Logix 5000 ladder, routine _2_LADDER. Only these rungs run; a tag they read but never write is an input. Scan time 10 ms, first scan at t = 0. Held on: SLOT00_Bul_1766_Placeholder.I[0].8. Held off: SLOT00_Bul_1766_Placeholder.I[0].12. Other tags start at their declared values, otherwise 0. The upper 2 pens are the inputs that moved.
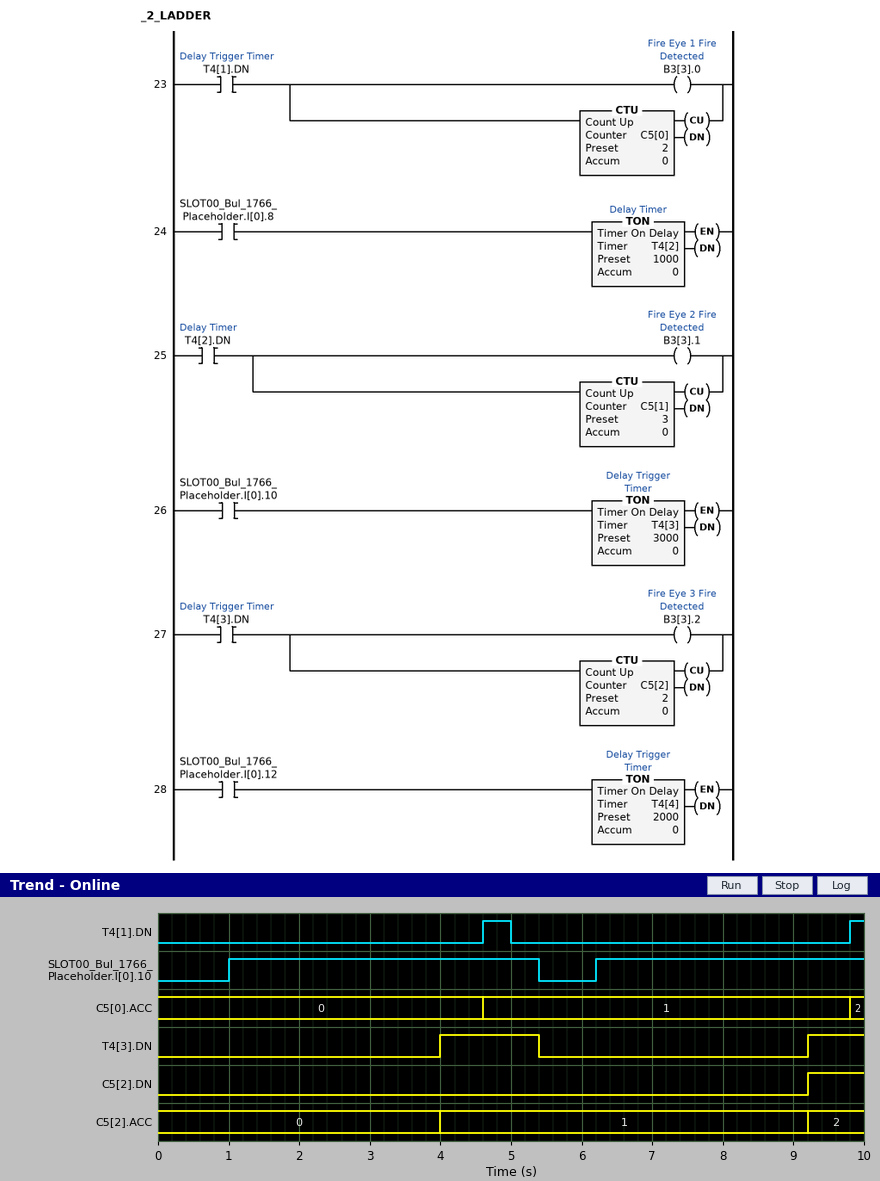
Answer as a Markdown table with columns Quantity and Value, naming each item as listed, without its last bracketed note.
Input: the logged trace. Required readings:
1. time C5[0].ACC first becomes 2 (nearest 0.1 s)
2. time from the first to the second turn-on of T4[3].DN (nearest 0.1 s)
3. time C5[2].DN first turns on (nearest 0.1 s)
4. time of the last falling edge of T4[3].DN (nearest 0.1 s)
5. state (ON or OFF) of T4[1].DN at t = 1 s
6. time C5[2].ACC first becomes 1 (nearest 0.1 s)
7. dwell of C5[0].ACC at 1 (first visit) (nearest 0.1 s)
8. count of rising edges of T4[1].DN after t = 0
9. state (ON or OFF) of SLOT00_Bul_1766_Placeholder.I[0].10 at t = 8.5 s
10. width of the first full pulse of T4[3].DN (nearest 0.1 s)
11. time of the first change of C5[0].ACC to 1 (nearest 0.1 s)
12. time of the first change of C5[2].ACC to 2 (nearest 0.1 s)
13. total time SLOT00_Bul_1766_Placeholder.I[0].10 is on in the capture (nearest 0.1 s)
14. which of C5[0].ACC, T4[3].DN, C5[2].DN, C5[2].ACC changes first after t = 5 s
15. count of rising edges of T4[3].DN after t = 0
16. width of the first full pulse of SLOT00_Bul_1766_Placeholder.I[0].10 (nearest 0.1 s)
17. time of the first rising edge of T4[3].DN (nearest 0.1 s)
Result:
| Quantity | Value |
|---|---|
| time C5[0].ACC first becomes 2 | 9.8 s |
| time from the first to the second turn-on of T4[3].DN | 5.2 s |
| time C5[2].DN first turns on | 9.2 s |
| time of the last falling edge of T4[3].DN | 5.4 s |
| state (ON or OFF) of T4[1].DN at t = 1 s | OFF |
| time C5[2].ACC first becomes 1 | 4.0 s |
| dwell of C5[0].ACC at 1 (first visit) | 5.2 s |
| count of rising edges of T4[1].DN after t = 0 | 2 |
| state (ON or OFF) of SLOT00_Bul_1766_Placeholder.I[0].10 at t = 8.5 s | ON |
| width of the first full pulse of T4[3].DN | 1.4 s |
| time of the first change of C5[0].ACC to 1 | 4.6 s |
| time of the first change of C5[2].ACC to 2 | 9.2 s |
| total time SLOT00_Bul_1766_Placeholder.I[0].10 is on in the capture | 8.2 s |
| which of C5[0].ACC, T4[3].DN, C5[2].DN, C5[2].ACC changes first after t = 5 s | T4[3].DN |
| count of rising edges of T4[3].DN after t = 0 | 2 |
| width of the first full pulse of SLOT00_Bul_1766_Placeholder.I[0].10 | 4.4 s |
| time of the first rising edge of T4[3].DN | 4.0 s |
